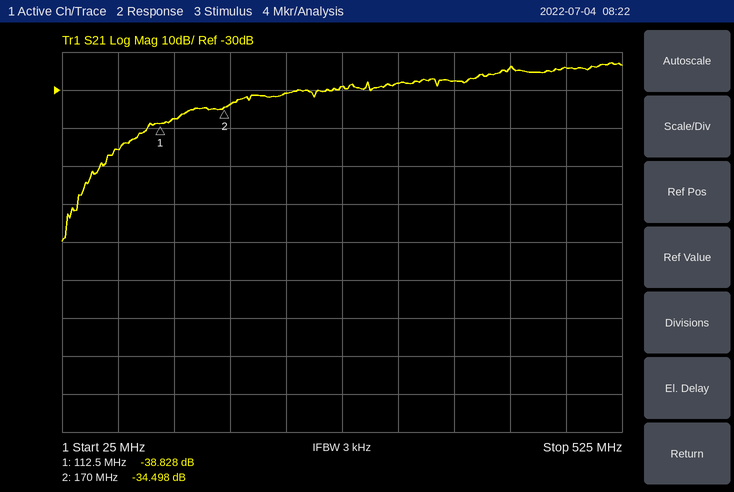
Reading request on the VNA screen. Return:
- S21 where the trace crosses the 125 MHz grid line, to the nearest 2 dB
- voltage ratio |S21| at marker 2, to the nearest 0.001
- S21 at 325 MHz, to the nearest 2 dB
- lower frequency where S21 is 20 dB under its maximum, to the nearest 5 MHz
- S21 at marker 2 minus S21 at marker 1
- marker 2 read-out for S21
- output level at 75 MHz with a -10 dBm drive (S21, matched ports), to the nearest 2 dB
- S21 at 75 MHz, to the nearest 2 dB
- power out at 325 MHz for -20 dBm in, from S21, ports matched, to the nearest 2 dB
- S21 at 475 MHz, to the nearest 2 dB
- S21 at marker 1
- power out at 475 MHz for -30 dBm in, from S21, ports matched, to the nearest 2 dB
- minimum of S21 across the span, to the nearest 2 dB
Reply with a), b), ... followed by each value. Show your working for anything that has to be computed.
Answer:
a) -38 dB
b) 10^(-34.498/20) ≈ 0.019
c) -28 dB
d) 90 MHz
e) -34.498 − (-38.828) = 4.330 dB
f) -34.498 dB
g) -10 dBm + (-46 dB) = -56 dBm
h) -46 dB
i) -20 dBm + (-28 dB) = -48 dBm
j) -24 dB
k) -38.828 dB
l) -30 dBm + (-24 dB) = -54 dBm
m) -70 dB
